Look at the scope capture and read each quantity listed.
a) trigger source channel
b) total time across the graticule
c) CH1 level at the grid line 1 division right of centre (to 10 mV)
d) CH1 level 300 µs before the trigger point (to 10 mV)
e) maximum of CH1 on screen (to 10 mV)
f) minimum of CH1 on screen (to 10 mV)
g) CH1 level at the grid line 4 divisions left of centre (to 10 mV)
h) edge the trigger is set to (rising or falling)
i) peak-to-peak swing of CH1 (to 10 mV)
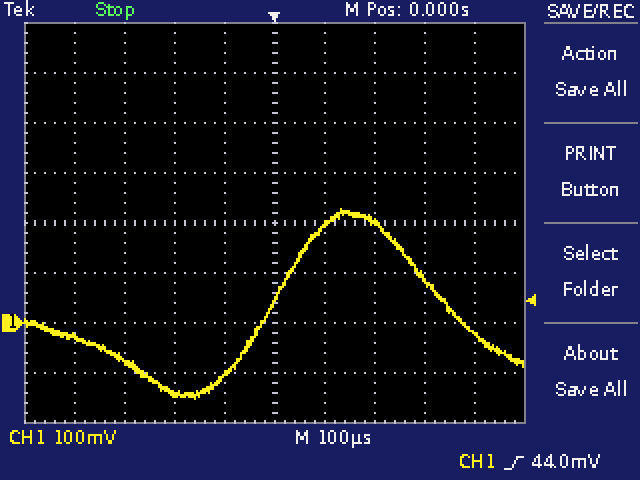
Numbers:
CH1
1 ms
190 mV
-80 mV
230 mV
-150 mV
-30 mV
rising
380 mV
